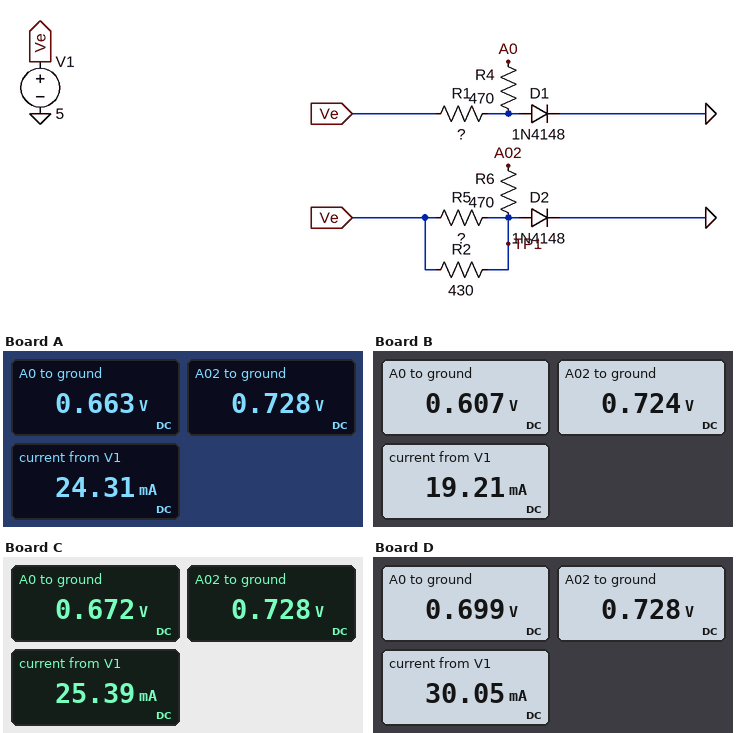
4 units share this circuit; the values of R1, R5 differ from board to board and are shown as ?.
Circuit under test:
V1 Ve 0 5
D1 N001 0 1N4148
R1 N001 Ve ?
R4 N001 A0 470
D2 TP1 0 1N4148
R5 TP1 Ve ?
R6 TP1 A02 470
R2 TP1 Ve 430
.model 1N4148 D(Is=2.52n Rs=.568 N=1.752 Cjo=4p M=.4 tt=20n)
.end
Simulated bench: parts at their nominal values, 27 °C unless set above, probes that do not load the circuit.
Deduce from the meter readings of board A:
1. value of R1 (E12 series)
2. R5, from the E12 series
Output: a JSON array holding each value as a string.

["820 Ω", "470 Ω"]
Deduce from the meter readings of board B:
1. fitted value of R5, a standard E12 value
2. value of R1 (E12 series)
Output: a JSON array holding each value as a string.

["560 Ω", "2.7 kΩ"]
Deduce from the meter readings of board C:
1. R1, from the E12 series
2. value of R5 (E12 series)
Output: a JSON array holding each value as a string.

["680 Ω", "470 Ω"]
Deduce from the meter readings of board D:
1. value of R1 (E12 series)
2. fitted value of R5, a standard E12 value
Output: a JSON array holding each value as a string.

["390 Ω", "470 Ω"]
